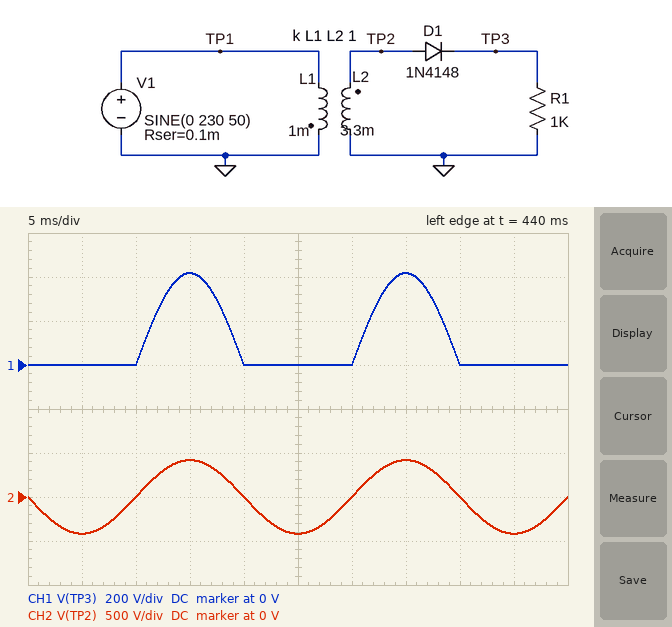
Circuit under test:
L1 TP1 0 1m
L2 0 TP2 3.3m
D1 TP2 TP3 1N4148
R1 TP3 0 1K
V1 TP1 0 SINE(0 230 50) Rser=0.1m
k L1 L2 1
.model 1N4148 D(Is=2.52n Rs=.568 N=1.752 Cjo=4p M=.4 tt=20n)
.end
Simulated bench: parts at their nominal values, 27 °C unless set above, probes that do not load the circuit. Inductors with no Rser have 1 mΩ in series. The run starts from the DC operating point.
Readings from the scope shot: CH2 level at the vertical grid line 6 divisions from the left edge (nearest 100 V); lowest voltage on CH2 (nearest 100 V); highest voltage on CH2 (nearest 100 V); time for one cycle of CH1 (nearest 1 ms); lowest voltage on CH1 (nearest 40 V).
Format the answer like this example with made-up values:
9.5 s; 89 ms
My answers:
0 V; -400 V; 400 V; 20 ms; 0 V
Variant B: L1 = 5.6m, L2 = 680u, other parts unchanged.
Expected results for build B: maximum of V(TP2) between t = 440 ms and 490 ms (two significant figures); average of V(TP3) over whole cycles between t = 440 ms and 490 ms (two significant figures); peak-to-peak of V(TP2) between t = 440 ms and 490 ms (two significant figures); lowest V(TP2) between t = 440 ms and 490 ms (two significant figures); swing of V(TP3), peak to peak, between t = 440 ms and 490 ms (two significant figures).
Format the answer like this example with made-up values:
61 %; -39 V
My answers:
80 V; 25 V; 160 V; -80 V; 79 V
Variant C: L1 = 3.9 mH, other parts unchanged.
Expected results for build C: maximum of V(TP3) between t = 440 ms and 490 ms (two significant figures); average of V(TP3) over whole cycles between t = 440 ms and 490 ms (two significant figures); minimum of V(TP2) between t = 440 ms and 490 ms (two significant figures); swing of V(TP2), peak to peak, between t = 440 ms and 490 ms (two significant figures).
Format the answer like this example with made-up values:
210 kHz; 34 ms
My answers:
210 V; 67 V; -210 V; 420 V
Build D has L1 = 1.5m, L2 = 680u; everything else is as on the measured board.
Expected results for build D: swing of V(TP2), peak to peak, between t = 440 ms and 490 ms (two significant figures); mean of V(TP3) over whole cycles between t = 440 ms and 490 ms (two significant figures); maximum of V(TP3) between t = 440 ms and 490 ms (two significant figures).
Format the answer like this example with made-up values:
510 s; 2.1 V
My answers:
310 V; 49 V; 150 V
